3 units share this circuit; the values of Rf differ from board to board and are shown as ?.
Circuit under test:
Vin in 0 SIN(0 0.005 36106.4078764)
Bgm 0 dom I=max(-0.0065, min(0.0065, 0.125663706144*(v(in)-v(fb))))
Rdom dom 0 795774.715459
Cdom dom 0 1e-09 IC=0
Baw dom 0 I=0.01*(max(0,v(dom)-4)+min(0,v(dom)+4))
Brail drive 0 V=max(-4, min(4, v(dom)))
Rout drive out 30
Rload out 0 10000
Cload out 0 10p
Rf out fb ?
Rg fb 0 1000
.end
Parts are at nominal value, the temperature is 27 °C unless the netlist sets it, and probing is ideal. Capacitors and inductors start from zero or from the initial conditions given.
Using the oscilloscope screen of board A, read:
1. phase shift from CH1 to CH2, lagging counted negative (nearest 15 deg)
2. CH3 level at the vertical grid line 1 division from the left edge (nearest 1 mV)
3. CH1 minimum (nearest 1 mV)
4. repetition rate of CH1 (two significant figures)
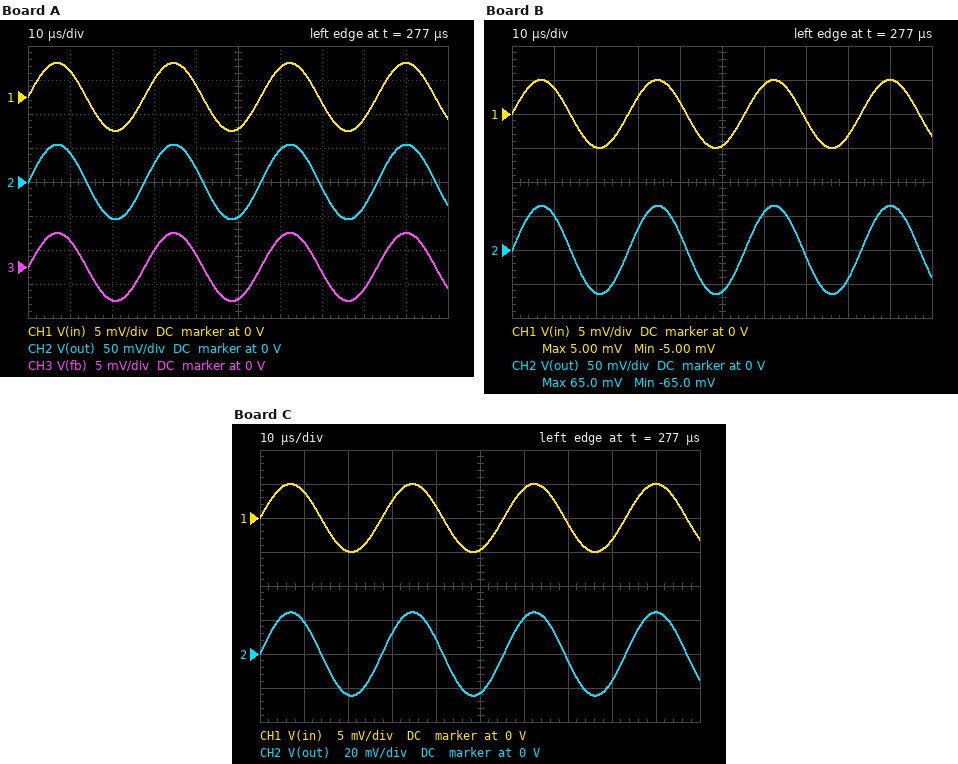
0 deg
4 mV
-5 mV
36 kHz
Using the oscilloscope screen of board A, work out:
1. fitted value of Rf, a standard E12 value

10 kΩ
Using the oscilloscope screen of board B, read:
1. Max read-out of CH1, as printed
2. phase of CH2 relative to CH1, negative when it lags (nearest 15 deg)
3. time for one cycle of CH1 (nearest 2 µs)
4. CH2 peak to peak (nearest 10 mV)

5.00 mV
0 deg
28 µs
130 mV
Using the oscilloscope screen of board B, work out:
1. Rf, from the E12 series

12 kΩ
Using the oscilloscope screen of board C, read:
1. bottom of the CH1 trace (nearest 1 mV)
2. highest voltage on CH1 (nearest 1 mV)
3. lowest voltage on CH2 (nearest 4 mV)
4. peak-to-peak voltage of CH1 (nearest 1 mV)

-5 mV
5 mV
-24 mV
10 mV
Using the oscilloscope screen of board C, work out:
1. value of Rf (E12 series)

3.9 kΩ
